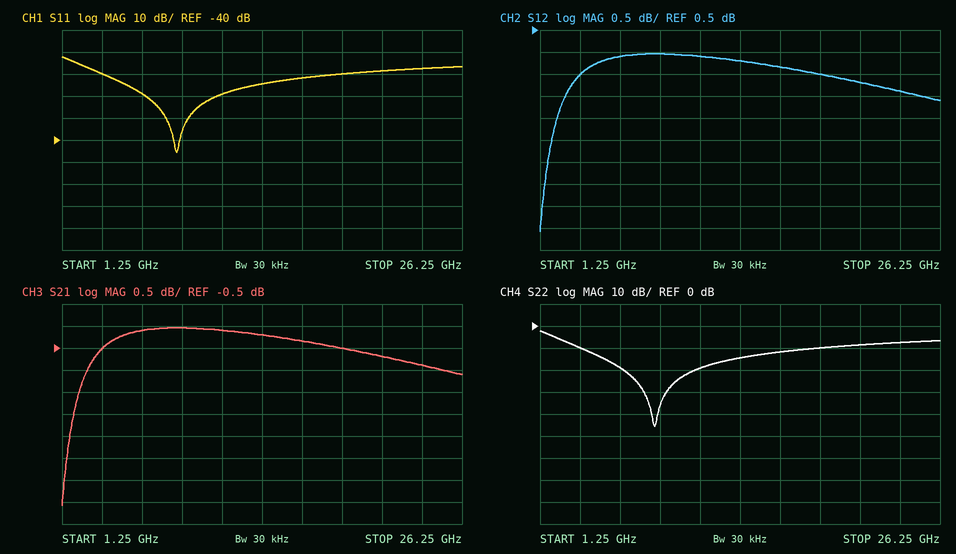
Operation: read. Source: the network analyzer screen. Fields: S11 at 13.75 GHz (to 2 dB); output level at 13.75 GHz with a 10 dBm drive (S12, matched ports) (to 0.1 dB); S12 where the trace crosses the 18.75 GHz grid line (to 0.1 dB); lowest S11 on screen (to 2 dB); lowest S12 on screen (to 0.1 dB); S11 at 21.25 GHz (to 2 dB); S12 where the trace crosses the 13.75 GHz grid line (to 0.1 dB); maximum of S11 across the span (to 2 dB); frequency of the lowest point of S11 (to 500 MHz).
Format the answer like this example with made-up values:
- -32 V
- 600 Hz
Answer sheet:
- -14 dB
- 9.8 dBm
- -0.5 dB
- -46 dB
- -4.1 dB
- -8 dB
- -0.2 dB
- -2 dB
- 8.5 GHz
